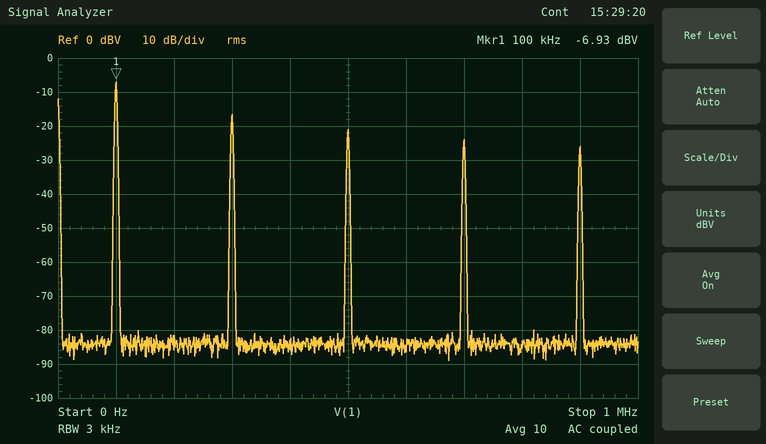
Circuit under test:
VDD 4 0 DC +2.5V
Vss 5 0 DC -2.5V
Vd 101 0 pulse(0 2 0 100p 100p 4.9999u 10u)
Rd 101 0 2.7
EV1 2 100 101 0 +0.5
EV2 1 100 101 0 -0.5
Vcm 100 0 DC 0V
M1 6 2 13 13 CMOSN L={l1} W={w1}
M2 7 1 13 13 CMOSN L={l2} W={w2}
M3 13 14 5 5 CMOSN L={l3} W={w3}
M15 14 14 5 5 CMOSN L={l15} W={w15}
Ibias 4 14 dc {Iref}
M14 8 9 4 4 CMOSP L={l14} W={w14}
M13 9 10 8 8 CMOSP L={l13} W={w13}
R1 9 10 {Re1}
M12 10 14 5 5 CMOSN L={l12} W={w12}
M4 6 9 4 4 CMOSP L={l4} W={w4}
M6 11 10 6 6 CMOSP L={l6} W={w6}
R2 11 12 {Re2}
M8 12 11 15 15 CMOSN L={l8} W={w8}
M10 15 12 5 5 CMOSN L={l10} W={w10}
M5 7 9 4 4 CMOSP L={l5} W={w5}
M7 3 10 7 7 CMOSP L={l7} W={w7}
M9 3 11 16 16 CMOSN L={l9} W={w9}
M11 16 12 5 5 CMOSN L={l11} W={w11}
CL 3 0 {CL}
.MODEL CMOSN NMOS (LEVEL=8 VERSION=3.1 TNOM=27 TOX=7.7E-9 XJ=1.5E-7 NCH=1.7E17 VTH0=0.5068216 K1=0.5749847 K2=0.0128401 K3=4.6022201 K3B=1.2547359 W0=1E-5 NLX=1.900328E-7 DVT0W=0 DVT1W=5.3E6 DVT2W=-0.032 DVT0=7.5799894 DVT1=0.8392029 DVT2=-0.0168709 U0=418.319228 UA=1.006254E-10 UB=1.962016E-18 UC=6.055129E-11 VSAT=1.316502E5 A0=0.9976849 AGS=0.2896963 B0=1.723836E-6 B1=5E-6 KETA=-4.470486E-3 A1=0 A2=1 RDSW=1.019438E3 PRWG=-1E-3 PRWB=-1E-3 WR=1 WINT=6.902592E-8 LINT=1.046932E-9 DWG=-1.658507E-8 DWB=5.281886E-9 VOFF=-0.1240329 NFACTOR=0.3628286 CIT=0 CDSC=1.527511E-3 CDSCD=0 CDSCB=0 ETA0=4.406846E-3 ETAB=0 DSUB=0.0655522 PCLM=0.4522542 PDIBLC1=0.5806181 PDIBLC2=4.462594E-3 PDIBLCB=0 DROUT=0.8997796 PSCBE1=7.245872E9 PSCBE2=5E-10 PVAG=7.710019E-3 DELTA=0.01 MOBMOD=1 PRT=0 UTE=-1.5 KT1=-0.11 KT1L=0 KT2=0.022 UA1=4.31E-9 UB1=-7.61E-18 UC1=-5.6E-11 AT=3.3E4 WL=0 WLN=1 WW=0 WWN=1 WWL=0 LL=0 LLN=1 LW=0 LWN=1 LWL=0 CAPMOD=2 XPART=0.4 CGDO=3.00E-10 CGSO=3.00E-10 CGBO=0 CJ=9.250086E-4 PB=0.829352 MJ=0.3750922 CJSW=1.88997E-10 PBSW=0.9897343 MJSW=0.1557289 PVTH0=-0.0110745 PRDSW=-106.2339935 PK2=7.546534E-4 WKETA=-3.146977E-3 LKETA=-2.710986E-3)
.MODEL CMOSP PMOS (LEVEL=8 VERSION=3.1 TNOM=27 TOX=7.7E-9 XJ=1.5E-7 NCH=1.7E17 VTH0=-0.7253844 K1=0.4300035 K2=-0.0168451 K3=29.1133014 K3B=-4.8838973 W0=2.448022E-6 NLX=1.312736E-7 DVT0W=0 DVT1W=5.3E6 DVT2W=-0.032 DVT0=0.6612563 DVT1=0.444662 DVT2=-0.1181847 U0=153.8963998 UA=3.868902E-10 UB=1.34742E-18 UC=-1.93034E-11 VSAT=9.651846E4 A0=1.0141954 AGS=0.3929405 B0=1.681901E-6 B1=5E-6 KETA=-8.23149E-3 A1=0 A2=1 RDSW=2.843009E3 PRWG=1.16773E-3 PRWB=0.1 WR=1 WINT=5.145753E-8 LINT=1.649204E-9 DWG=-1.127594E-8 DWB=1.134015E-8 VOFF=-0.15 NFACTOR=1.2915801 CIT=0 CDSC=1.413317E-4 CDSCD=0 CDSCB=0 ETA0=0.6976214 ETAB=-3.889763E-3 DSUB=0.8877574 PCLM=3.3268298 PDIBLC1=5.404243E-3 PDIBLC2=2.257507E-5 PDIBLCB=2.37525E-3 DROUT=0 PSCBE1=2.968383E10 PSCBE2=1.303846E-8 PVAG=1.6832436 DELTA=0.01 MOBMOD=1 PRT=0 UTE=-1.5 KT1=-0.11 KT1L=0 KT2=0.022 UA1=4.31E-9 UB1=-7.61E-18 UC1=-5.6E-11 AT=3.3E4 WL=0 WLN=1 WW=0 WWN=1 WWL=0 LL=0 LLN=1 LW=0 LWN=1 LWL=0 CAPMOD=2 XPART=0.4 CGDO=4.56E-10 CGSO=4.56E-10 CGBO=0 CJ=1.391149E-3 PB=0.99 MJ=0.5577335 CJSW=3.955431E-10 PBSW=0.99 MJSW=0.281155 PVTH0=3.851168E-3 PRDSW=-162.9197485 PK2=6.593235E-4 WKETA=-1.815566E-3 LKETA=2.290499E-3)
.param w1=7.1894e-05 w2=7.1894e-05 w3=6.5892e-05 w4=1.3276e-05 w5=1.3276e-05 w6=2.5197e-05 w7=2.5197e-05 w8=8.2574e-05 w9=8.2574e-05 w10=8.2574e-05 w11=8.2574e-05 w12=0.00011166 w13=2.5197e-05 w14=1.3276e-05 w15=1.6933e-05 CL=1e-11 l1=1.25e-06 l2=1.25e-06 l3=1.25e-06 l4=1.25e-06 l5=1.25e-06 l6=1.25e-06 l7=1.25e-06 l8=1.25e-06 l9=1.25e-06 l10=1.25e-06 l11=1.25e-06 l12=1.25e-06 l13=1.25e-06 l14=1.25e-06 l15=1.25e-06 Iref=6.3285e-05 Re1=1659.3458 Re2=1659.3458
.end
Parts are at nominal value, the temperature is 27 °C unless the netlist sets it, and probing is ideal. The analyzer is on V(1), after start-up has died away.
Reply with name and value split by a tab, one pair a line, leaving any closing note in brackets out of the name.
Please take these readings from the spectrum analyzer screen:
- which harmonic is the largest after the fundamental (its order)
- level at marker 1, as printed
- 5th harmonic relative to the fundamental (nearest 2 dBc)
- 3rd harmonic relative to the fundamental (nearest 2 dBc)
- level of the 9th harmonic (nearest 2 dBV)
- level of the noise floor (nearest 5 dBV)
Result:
which harmonic is the largest after the fundamental	3
level at marker 1, as printed	-6.93 dBV
5th harmonic relative to the fundamental	-14 dBc
3rd harmonic relative to the fundamental	-10 dBc
level of the 9th harmonic	-26 dBV
level of the noise floor	-85 dBV
